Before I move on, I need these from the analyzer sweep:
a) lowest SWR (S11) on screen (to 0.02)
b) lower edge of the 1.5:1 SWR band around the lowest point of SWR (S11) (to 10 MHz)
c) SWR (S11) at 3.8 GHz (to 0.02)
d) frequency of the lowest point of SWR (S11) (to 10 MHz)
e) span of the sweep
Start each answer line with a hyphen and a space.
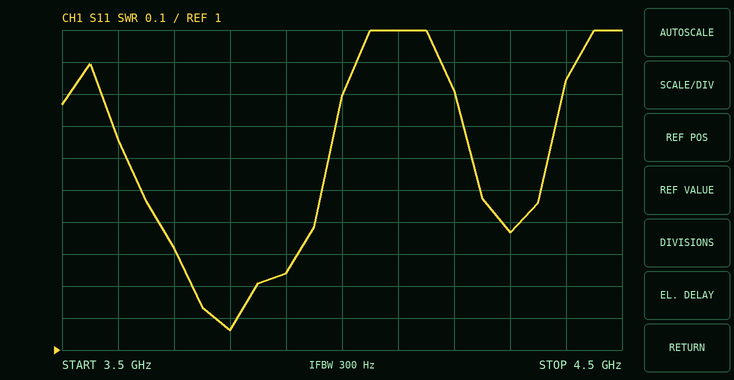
- 1.06
- 3.64 GHz
- 1.06
- 3.80 GHz
- 1 GHz
